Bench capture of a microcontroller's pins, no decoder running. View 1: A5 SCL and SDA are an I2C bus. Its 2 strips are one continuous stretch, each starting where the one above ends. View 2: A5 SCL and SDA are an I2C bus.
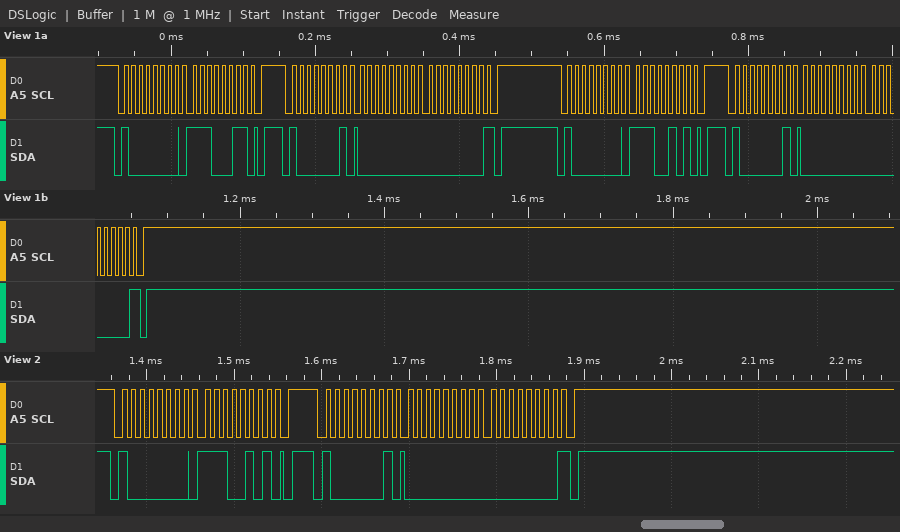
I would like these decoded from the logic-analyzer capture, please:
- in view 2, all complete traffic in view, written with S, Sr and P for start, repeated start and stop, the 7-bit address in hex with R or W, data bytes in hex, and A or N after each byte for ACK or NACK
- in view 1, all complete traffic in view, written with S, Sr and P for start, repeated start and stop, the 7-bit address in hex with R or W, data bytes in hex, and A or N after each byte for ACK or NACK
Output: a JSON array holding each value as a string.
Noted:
["S 40W A E5 A P S 40R A 00 A 00 N P", "S 40W A E3 A P S 40R A 00 A 00 N P S 40W A E5 A P S 40R A 00 A 00 N P"]
